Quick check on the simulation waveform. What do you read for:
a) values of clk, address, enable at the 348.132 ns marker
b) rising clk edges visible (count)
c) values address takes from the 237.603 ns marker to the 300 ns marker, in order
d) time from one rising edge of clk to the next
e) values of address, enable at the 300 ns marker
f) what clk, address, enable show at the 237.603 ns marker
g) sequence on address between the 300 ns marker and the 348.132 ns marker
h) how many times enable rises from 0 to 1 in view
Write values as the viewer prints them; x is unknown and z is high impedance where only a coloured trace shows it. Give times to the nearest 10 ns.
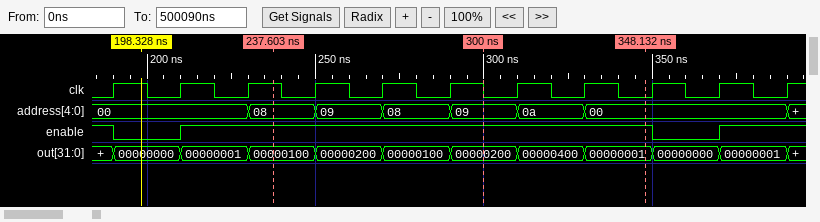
clk=0, address=00, enable=1
11
08, 09, 08, 09
20 ns
address=09, enable=1
clk=1, address=08, enable=1
09, 0a, 00
2
